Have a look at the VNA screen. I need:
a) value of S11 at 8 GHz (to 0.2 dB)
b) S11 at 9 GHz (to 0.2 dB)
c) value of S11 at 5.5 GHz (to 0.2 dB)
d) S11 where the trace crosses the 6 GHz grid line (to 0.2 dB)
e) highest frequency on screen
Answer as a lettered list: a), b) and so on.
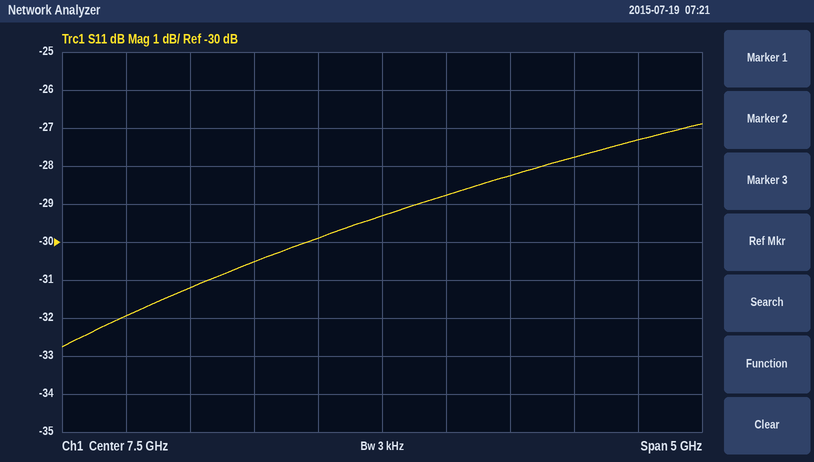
a) -28.8 dB
b) -27.8 dB
c) -32.0 dB
d) -31.2 dB
e) 10 GHz
